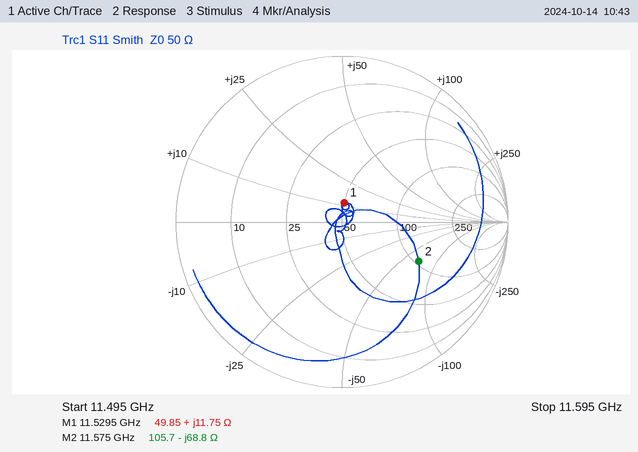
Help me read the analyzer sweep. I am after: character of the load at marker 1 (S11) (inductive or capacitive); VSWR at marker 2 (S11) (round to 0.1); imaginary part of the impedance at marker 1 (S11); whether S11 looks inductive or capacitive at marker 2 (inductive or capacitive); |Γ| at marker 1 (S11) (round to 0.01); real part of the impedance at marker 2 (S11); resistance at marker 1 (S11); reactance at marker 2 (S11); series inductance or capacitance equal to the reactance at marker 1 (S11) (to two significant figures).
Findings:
inductive
3.2
+11.75 Ω
capacitive
0.12
105.7 Ω
49.85 Ω
-68.8 Ω
160 pH
